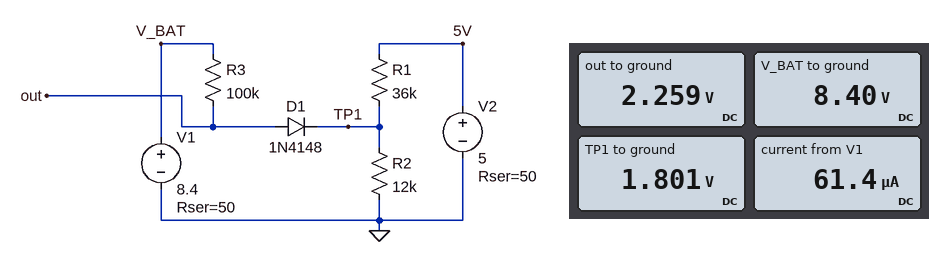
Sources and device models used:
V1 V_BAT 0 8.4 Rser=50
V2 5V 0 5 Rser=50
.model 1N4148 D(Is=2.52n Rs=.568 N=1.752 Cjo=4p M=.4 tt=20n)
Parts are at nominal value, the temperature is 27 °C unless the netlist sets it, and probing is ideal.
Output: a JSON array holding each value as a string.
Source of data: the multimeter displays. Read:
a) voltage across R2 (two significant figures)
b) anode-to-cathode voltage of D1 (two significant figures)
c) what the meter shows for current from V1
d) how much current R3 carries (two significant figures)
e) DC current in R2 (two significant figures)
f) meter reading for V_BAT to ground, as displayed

["1.8 V", "460 mV", "61.4 µA", "61 µA", "150 µA", "8.40 V"]
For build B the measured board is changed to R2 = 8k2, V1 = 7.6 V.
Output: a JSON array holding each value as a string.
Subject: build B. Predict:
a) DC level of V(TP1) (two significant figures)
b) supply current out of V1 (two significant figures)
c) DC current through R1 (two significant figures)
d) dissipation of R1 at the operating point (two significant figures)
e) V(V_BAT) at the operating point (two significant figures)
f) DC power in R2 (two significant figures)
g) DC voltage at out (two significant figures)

["1.3 V", "58 µA", "100 µA", "380 µW", "7.6 V", "210 µW", "1.8 V"]
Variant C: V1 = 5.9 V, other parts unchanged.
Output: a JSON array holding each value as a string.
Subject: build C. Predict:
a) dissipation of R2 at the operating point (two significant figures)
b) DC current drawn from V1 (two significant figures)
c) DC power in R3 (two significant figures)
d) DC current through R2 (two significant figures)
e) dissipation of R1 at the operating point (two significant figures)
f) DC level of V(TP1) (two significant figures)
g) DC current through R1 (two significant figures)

["210 µW", "39 µA", "150 µW", "130 µA", "320 µW", "1.6 V", "94 µA"]
